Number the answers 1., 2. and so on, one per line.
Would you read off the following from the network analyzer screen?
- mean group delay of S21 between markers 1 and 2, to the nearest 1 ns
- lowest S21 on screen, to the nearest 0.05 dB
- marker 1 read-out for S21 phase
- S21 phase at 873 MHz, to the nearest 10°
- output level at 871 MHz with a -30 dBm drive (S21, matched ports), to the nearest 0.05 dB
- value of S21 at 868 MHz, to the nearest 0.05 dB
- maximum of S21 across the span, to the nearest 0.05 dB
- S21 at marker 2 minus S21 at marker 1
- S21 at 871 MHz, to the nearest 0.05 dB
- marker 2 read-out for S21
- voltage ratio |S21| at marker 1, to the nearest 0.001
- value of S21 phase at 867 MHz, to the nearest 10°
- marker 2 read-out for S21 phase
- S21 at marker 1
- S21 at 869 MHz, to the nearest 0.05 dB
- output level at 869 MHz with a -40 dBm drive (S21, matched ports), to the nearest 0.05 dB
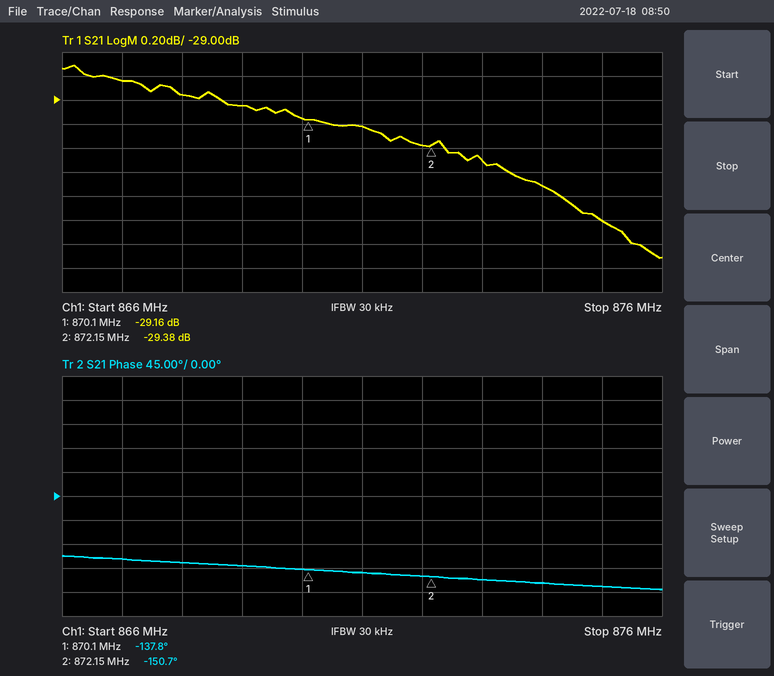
1. 17 ns
2. -30.30 dB
3. -137.8°
4. -160°
5. -59.20 dBm
6. -28.95 dB
7. -28.70 dB
8. -0.22 dB
9. -29.20 dB
10. -29.38 dB
11. 0.035
12. -120°
13. -150.7°
14. -29.16 dB
15. -29.05 dB
16. -69.05 dBm
